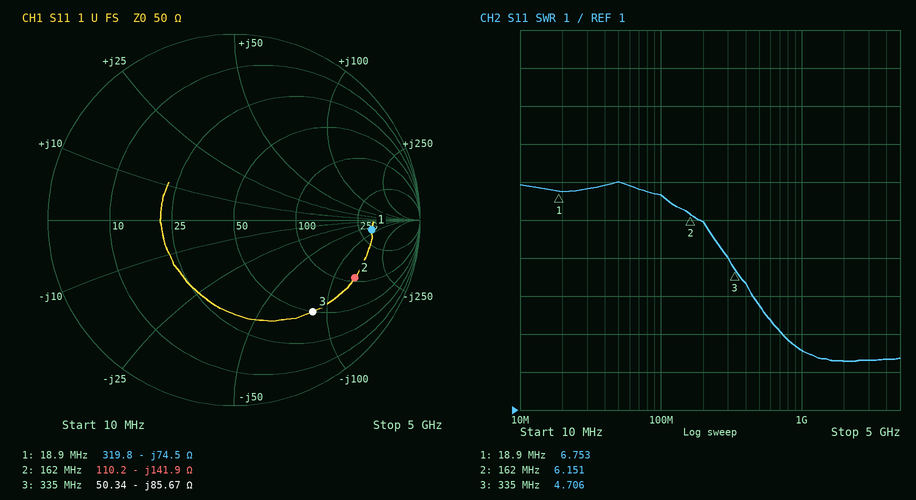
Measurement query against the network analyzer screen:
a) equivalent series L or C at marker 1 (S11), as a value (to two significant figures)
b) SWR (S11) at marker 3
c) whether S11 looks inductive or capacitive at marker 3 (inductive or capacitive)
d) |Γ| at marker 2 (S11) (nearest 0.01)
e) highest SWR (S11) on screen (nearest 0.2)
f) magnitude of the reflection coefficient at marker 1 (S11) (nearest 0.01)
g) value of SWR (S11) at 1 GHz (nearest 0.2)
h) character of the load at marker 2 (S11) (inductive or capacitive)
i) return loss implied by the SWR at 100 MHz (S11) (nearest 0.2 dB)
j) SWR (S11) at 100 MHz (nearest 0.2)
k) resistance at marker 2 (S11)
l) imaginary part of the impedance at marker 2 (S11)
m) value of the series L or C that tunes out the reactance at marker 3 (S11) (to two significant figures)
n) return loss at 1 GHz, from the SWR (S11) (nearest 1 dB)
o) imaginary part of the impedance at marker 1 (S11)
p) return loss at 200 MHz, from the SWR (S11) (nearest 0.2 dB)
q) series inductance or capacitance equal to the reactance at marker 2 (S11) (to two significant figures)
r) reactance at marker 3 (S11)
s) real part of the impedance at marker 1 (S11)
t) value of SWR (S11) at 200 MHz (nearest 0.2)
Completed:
110 pF
4.706
capacitive
0.72
7.0
0.74
2.6
capacitive
2.6 dB
6.6
110.2 Ω
-141.9 Ω
41 nH
7 dB
-74.5 Ω
3.0 dB
6.9 pF
-85.67 Ω
319.8 Ω
6.0
